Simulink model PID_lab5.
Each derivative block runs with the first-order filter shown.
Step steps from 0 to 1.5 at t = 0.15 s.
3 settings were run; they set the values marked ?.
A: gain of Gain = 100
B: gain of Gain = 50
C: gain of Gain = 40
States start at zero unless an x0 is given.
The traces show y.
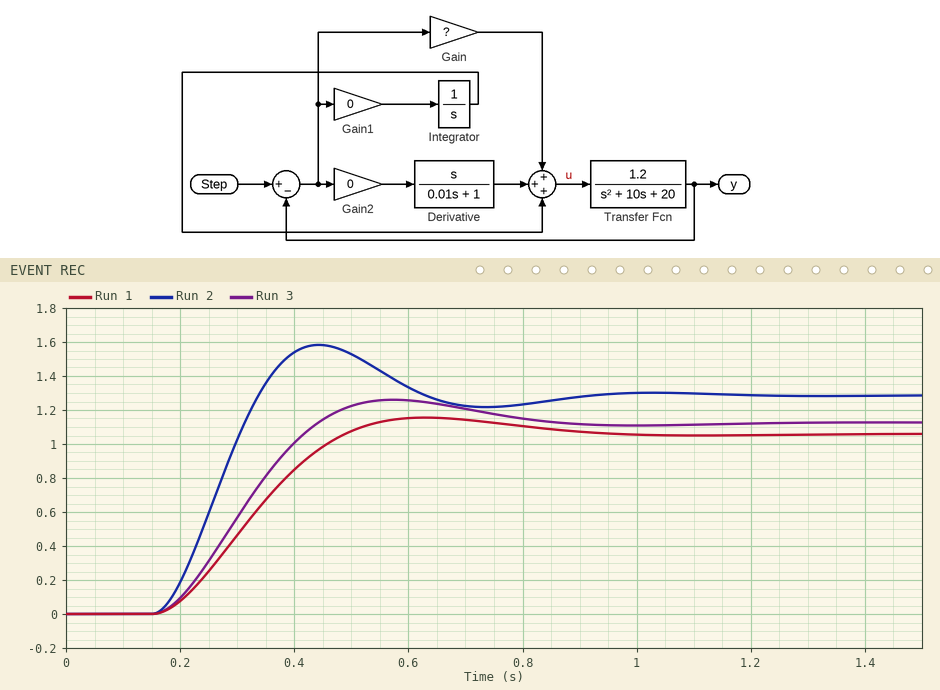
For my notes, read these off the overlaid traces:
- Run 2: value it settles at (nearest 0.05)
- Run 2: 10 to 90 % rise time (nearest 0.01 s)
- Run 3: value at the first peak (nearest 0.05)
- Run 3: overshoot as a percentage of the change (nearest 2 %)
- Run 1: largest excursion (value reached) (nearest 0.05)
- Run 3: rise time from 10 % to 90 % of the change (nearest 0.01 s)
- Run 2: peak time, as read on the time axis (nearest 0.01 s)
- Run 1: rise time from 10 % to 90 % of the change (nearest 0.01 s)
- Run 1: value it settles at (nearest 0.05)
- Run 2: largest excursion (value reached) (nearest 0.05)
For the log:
1.30
0.13 s
1.25
12 %
1.15
0.20 s
0.44 s
0.23 s
1.05
1.60
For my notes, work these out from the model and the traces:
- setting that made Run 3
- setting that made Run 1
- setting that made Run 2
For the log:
B
C
A
